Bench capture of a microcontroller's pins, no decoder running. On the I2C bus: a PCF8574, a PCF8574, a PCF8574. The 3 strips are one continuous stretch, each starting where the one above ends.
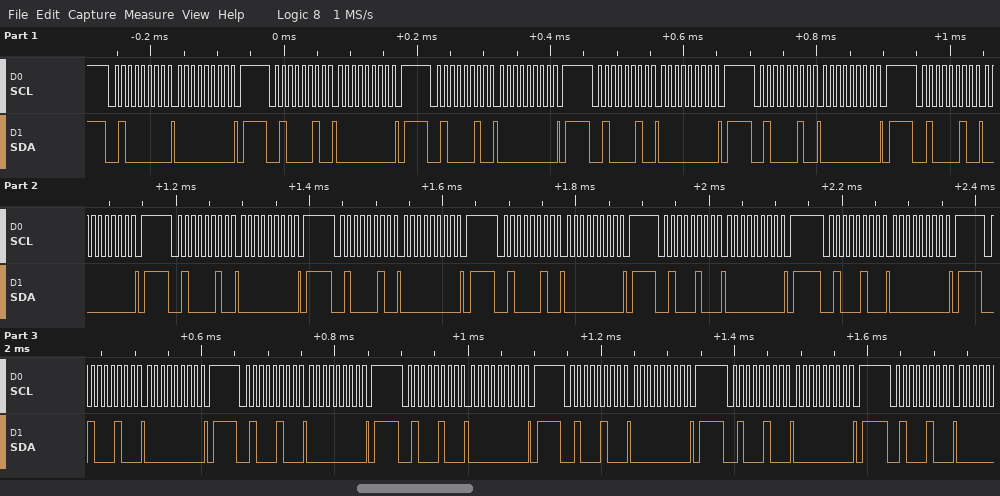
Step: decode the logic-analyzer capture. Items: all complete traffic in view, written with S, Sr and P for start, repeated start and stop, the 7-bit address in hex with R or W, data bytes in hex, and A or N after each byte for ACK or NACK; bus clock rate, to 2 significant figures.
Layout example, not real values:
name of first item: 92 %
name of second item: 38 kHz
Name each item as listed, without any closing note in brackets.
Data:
all complete traffic in view, written with S, Sr and P for start, repeated start and stop, the 7-bit address in hex with R or W, data bytes in hex, and A or N after each byte for ACK or NACK: S 20W A 00 A P S 21W A 00 A P S 21W A 00 A P S 21W A 00 A P S 21W A 00 A P S 21W A 00 A P S 21W A 00 A P S 21W A 00 A P S 21W A 00 A P S 22W A 00 A P S 22W A 00 A P S 22W A 00 A P S 22W A 00 A P S 22W A 00 A P S 22W A 00 A P S 22W A 00 A P S 22W A
bus clock rate, to 2 significant figures: 100 kHz
